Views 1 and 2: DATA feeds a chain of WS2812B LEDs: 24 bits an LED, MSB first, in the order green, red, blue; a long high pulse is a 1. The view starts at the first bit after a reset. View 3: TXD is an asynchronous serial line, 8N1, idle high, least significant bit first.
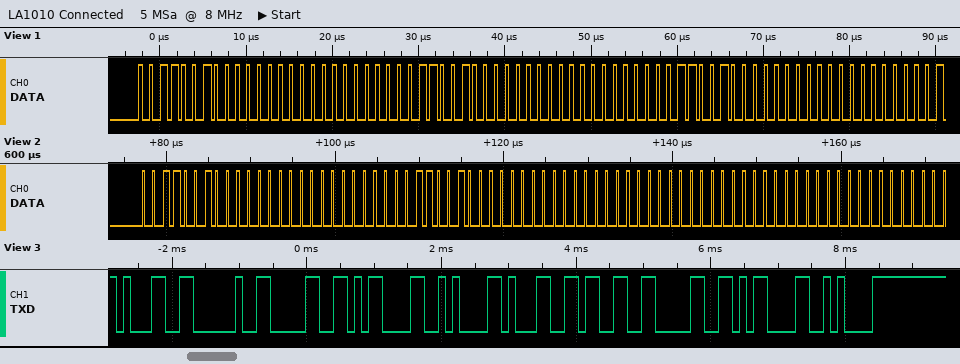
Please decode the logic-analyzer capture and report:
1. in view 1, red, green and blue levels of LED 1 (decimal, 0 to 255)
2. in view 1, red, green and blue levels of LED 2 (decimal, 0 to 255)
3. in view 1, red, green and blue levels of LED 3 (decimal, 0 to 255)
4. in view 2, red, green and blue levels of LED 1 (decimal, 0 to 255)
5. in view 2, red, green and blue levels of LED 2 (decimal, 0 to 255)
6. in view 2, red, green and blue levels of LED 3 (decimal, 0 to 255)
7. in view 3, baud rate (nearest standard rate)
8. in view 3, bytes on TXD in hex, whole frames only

0, 50, 0
0, 50, 0
0, 50, 0
0, 50, 0
0, 50, 0
0, 0, 0
9600 baud
31 20 30 0D 0A 31 33 30 0D 0A
